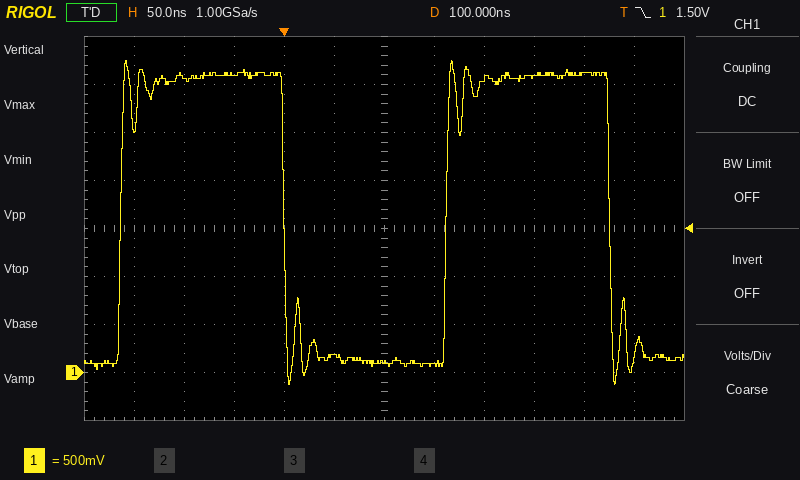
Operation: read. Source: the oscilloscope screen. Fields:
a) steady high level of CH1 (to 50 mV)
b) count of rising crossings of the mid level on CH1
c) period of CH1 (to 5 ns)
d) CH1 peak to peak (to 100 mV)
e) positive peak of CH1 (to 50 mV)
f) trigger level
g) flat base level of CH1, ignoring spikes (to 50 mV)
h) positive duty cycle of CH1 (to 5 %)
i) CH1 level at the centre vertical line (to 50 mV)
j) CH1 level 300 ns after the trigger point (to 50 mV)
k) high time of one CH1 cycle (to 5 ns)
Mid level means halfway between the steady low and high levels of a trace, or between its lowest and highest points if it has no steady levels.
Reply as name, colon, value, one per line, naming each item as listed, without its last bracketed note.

steady high level of CH1: 3.10 V
count of rising crossings of the mid level on CH1: 2
period of CH1: 325 ns
CH1 peak to peak: 3.40 V
positive peak of CH1: 3.25 V
trigger level: 1.50 V
flat base level of CH1, ignoring spikes: 100 mV
positive duty cycle of CH1: 50 %
CH1 level at the centre vertical line: 100 mV
CH1 level 300 ns after the trigger point: 3.10 V
high time of one CH1 cycle: 165 ns
